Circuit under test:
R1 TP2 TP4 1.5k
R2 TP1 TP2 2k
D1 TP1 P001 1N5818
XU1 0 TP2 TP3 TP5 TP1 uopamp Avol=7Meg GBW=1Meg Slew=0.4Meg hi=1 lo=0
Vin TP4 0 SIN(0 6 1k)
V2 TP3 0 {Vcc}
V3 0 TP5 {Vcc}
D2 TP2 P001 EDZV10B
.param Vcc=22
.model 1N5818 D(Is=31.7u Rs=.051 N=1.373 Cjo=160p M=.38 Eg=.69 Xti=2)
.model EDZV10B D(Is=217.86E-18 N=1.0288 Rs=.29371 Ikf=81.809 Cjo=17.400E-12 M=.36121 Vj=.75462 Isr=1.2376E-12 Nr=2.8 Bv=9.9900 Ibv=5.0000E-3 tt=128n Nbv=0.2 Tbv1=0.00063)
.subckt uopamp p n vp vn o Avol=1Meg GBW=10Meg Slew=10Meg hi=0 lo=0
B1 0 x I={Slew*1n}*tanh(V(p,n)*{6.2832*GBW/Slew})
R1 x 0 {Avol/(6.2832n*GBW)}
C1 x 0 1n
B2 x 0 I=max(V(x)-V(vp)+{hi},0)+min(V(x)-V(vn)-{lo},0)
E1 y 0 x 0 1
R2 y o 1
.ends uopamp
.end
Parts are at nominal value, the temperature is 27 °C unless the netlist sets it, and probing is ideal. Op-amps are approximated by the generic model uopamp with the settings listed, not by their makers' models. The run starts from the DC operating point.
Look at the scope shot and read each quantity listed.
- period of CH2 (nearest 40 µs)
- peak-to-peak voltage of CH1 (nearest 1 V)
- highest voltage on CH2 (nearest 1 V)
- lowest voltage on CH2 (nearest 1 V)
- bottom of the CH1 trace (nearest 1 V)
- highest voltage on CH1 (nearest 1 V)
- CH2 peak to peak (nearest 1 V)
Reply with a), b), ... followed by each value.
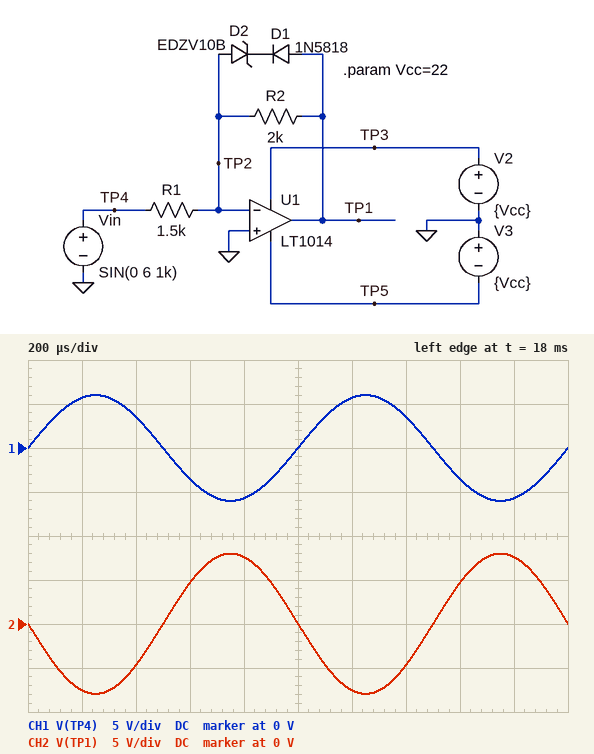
a) 1.00 ms
b) 12 V
c) 8 V
d) -8 V
e) -6 V
f) 6 V
g) 16 V
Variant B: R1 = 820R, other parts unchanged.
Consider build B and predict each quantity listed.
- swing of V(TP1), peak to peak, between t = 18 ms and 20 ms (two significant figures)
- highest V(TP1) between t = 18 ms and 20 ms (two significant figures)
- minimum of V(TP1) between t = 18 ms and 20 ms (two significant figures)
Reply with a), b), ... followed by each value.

a) 25 V
b) 10 V
c) -15 V
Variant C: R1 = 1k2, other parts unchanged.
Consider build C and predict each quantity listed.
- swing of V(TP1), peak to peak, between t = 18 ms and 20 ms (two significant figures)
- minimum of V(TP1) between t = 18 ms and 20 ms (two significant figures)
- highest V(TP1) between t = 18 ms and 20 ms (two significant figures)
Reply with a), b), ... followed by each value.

a) 20 V
b) -9.9 V
c) 10 V
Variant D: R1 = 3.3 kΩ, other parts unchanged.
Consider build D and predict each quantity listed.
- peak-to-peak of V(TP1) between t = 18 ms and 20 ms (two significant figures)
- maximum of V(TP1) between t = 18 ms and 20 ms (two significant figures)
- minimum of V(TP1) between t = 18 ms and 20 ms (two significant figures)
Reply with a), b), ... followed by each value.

a) 7.2 V
b) 3.6 V
c) -3.6 V
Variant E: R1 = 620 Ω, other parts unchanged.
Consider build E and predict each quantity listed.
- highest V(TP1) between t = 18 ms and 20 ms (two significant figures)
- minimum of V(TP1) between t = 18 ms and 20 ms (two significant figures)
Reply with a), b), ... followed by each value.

a) 10 V
b) -19 V
